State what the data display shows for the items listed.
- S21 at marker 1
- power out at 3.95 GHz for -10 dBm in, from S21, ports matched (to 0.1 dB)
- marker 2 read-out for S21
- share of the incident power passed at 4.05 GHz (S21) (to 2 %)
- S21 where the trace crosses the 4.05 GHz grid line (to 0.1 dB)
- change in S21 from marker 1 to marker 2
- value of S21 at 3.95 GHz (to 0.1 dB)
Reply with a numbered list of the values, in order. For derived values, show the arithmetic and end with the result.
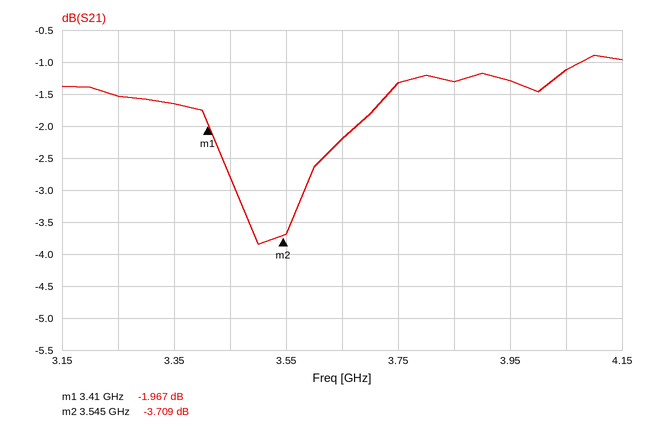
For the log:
1. -1.967 dB
2. -10 dBm + (-1.3 dB) = -11.3 dBm
3. -3.709 dB
4. 10^(-1.1/10) ≈ 78 %
5. -1.1 dB
6. -3.709 − (-1.967) = -1.742 dB
7. -1.3 dB
